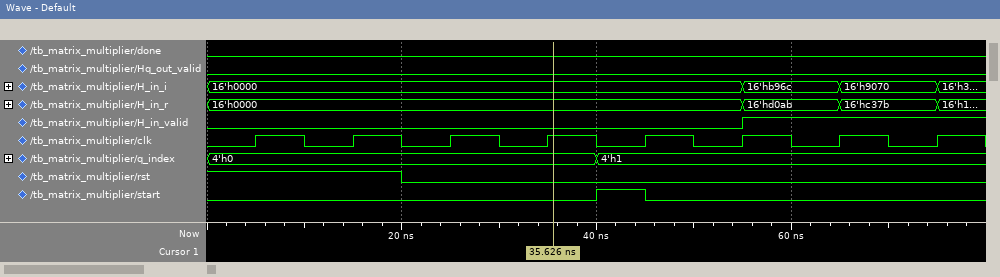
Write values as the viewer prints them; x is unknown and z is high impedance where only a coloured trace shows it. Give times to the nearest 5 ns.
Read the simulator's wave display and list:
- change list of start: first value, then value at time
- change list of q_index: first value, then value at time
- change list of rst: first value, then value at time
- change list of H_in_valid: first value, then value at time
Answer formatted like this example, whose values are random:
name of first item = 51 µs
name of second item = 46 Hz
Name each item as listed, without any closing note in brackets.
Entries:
change list of start: first value, then value at time = 0, 1 at 40 ns, 0 at 45 ns
change list of q_index: first value, then value at time = 4'h0, 4'h1 at 40 ns
change list of rst: first value, then value at time = 1, 0 at 20 ns
change list of H_in_valid: first value, then value at time = 0, 1 at 55 ns
